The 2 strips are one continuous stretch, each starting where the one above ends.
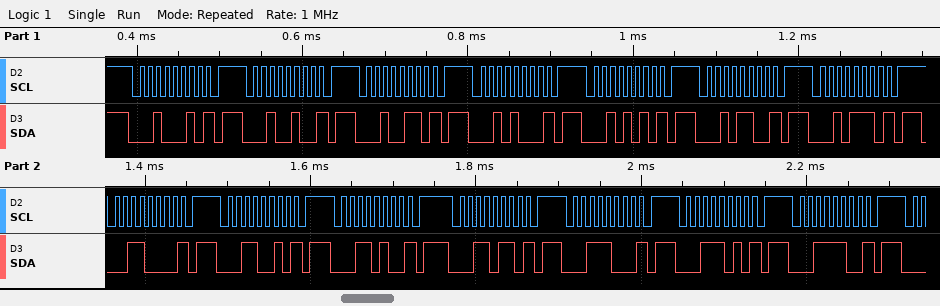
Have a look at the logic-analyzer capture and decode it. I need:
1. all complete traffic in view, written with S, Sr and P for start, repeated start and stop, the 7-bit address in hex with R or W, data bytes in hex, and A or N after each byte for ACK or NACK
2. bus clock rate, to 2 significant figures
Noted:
S 11W N P S 12W N P S 13W N P S 14W N P S 15W N P S 16W N P S 17W N P S 18W N P S 19W N P S 1AW N P S 1BW N P S 1CW N P S 1DW N P S 1EW N P
100 kHz
